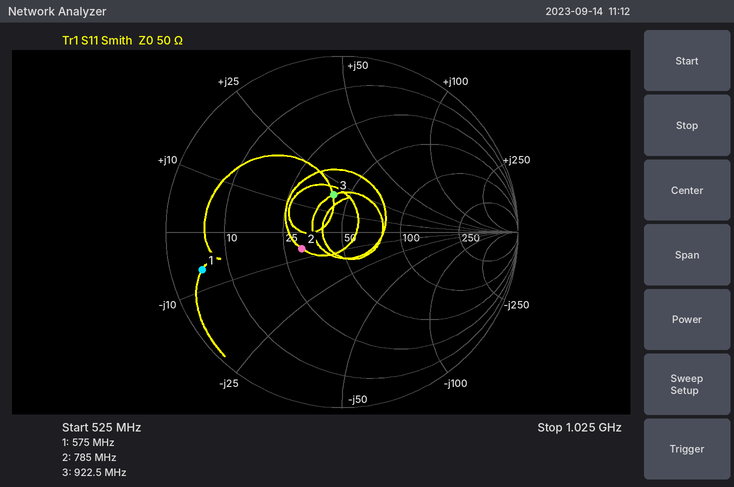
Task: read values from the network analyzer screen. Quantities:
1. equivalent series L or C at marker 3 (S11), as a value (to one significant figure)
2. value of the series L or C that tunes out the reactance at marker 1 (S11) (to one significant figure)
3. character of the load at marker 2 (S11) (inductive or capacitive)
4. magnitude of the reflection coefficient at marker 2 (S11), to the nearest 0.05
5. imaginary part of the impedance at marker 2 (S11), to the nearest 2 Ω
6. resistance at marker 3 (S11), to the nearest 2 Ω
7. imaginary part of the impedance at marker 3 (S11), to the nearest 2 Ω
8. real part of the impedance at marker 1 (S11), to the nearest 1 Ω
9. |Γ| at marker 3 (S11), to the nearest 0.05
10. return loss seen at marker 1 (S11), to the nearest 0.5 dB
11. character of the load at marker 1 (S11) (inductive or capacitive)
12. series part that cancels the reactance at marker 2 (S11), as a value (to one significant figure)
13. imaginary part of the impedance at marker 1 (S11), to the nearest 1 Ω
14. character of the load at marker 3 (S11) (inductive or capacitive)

3 nH
2 nH
capacitive
0.25
-6 Ω
42 Ω
+18 Ω
5 Ω
0.20
1.5 dB
capacitive
1 nH
-7 Ω
inductive
